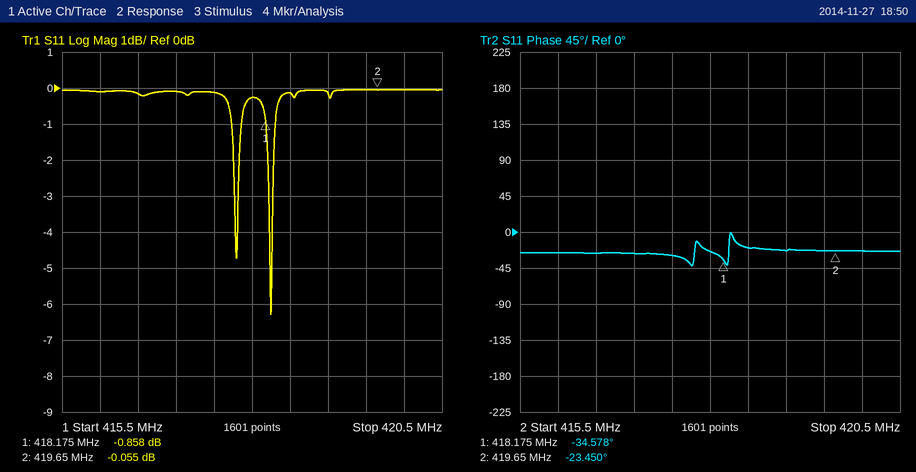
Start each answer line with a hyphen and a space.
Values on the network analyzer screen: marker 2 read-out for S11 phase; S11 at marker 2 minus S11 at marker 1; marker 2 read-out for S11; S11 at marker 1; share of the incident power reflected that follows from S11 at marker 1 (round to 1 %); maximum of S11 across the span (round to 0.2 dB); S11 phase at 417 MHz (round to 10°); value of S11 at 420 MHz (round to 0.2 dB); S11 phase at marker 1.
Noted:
- -23.450°
- 0.803 dB
- -0.055 dB
- -0.858 dB
- 82 %
- 0.0 dB
- -30°
- 0.0 dB
- -34.578°
